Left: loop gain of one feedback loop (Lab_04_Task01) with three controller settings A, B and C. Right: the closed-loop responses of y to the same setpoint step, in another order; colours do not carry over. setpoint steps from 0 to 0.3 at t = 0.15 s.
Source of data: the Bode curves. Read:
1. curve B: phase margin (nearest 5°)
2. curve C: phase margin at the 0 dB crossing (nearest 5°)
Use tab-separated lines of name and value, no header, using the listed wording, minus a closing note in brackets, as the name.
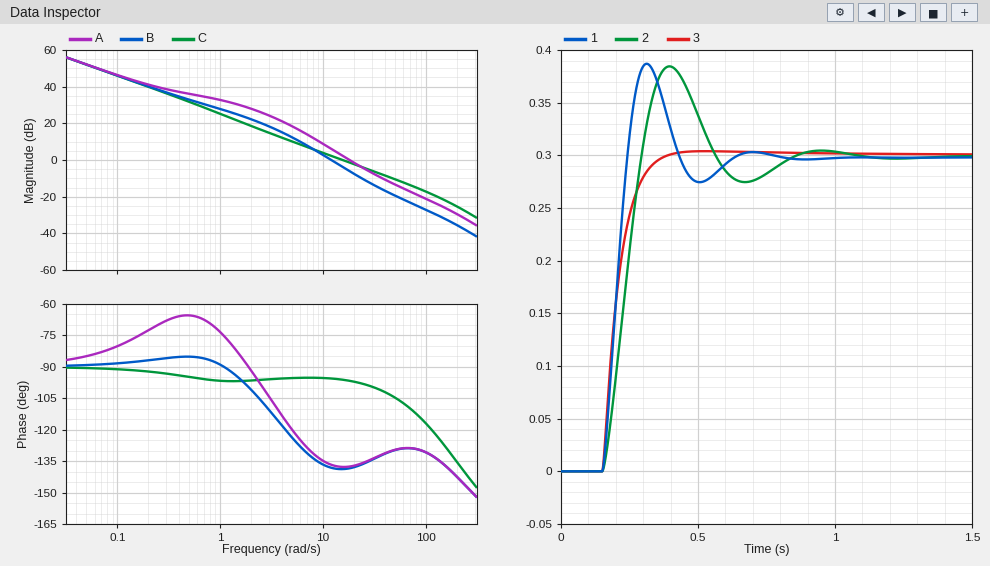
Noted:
curve B: phase margin	40°
curve C: phase margin at the 0 dB crossing	85°
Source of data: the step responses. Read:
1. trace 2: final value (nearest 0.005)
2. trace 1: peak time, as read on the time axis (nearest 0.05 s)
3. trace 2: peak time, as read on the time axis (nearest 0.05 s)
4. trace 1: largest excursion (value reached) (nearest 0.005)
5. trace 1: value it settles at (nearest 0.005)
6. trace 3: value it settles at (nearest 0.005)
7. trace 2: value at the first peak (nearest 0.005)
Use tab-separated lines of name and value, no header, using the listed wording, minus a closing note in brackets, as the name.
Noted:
trace 2: final value	0.300
trace 1: peak time, as read on the time axis	0.30 s
trace 2: peak time, as read on the time axis	0.40 s
trace 1: largest excursion (value reached)	0.385
trace 1: value it settles at	0.300
trace 3: value it settles at	0.300
trace 2: value at the first peak	0.385
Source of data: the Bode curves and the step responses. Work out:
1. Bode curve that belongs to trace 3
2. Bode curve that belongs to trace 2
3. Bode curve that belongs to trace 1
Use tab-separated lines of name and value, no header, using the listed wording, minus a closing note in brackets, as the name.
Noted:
Bode curve that belongs to trace 3	C
Bode curve that belongs to trace 2	B
Bode curve that belongs to trace 1	A
